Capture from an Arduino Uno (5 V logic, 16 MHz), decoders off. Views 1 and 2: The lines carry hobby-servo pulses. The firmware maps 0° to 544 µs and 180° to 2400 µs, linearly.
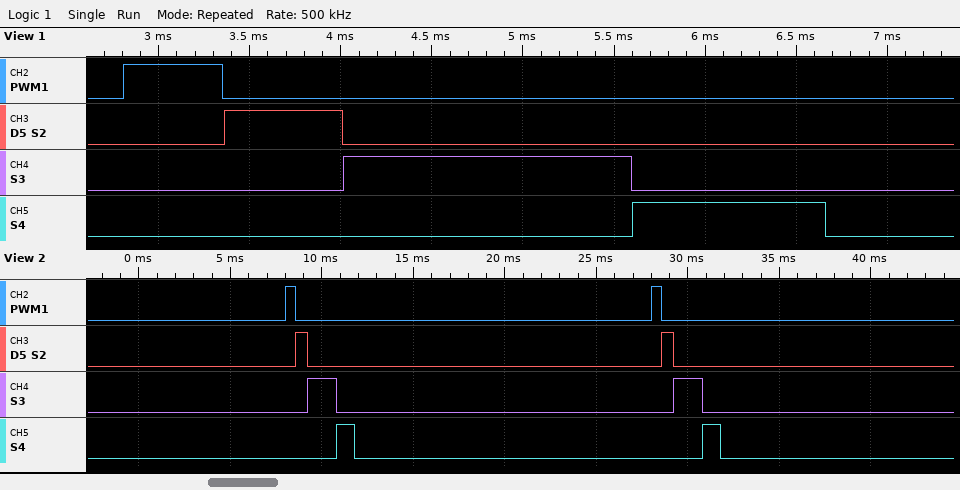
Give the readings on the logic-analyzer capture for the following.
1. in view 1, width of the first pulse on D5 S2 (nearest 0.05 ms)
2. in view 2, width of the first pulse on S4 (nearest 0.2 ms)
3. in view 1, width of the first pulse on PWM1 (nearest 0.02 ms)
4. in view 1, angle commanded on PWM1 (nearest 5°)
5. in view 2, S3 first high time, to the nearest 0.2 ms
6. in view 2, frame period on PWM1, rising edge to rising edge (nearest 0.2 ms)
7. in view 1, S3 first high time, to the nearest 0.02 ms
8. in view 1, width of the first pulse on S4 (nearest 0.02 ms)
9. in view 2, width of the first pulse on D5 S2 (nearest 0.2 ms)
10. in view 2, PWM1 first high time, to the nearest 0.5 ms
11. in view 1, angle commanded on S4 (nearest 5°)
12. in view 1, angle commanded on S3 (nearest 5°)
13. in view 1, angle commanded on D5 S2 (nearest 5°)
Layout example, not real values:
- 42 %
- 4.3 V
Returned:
- 0.65 ms
- 1.0 ms
- 0.54 ms
- 0°
- 1.6 ms
- 20.0 ms
- 1.58 ms
- 1.06 ms
- 0.6 ms
- 0.5 ms
- 50°
- 100°
- 10°
